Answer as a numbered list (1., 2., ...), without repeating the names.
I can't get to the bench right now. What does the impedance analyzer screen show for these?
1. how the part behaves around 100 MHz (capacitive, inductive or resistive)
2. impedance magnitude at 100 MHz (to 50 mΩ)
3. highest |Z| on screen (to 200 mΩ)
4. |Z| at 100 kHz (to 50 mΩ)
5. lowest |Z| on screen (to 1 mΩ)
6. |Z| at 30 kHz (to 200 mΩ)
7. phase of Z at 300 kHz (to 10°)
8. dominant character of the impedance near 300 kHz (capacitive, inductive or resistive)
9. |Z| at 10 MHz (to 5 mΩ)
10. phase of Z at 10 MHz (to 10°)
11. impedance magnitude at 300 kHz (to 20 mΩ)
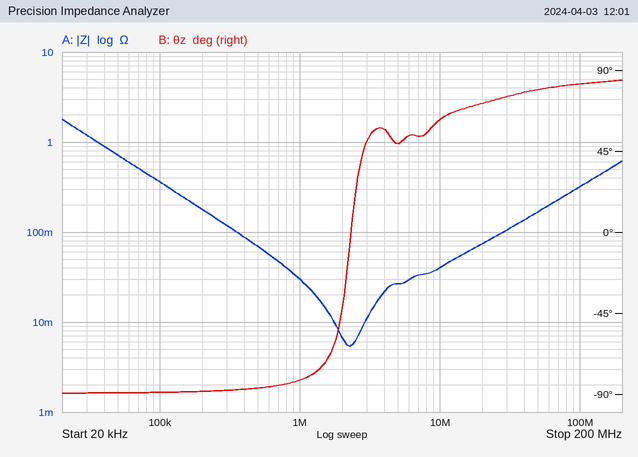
1. inductive
2. 300 mΩ
3. 1.8 Ω
4. 350 mΩ
5. 5 mΩ
6. 1.2 Ω
7. -90°
8. capacitive
9. 40 mΩ
10. 60°
11. 120 mΩ
